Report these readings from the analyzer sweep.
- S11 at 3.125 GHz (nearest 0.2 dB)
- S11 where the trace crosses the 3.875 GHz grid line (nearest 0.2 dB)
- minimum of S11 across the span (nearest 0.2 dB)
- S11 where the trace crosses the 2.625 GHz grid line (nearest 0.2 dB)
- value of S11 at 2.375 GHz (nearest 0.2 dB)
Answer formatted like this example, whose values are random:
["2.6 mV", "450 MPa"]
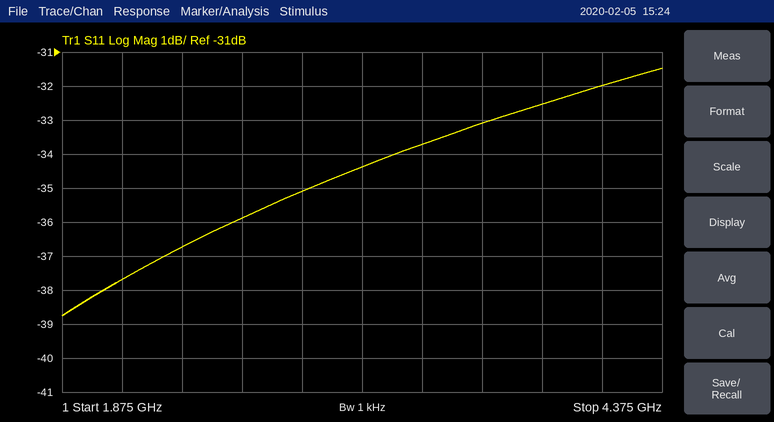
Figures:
["-34.4 dB", "-32.6 dB", "-38.8 dB", "-35.8 dB", "-36.8 dB"]
